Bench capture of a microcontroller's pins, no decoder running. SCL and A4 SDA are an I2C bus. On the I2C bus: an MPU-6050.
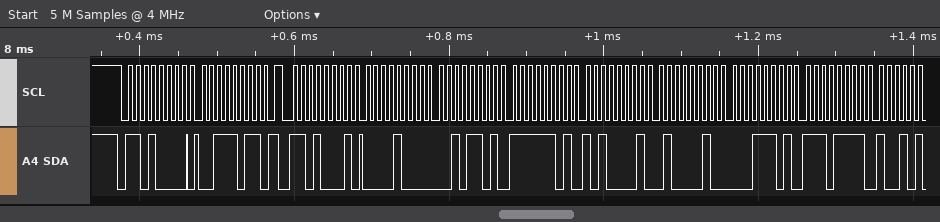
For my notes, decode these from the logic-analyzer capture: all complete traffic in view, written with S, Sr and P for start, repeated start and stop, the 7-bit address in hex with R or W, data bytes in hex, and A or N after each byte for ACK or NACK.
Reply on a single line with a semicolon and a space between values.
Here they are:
S 68W A 3B A Sr 68R A 08 A 2D A FD A A1 A 42 A 1D A EF A
